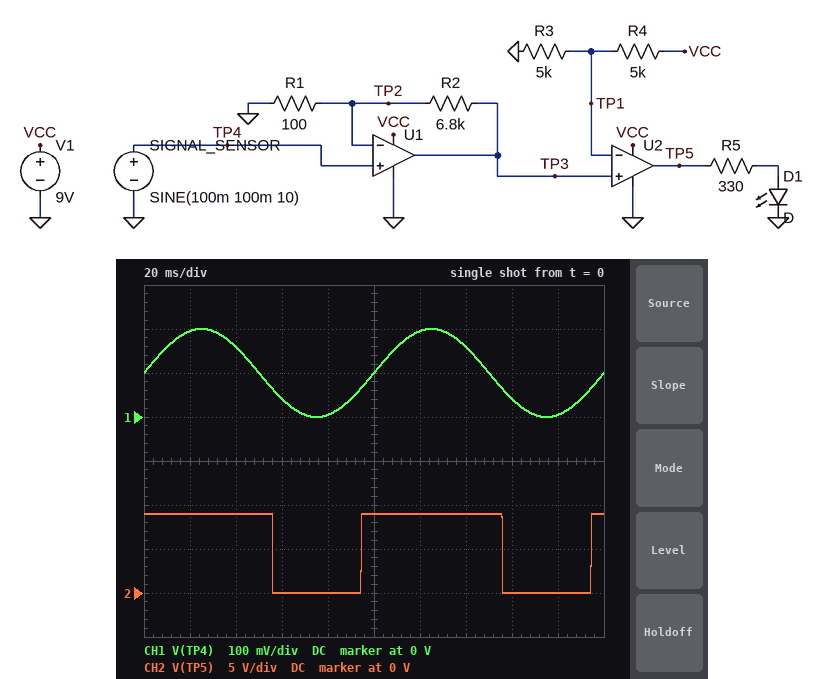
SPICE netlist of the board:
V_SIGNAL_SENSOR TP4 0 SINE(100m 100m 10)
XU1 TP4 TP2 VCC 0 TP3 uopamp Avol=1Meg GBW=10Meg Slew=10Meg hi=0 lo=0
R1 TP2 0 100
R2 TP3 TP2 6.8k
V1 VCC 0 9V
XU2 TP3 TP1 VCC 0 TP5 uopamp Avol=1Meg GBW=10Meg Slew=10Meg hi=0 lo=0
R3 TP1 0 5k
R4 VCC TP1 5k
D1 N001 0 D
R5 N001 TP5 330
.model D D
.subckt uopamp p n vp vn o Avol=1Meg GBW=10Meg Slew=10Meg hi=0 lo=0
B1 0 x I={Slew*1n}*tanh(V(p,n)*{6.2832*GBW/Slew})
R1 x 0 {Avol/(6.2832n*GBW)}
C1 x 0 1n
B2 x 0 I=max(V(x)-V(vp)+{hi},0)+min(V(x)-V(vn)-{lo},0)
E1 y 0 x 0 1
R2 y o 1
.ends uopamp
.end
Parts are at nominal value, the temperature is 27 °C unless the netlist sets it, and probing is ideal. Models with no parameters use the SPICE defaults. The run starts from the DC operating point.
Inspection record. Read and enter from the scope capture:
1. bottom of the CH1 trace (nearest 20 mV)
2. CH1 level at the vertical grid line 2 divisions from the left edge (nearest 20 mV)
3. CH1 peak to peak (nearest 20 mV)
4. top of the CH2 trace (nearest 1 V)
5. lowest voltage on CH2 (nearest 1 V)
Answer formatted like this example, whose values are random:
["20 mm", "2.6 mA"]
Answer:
["0 V", "160 mV", "200 mV", "9 V", "0 V"]
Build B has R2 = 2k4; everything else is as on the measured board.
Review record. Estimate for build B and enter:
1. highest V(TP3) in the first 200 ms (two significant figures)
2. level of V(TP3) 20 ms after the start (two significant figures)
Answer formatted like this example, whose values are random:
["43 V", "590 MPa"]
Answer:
["5.0 V", "4.9 V"]
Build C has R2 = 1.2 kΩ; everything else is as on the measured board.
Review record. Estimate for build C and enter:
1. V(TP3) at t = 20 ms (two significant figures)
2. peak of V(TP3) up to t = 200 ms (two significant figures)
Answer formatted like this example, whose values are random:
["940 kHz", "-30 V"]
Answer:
["2.5 V", "2.6 V"]
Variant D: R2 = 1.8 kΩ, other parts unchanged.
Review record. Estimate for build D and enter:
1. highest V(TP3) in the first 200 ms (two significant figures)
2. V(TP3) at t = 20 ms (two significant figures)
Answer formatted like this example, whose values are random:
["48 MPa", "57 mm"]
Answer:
["3.8 V", "3.7 V"]
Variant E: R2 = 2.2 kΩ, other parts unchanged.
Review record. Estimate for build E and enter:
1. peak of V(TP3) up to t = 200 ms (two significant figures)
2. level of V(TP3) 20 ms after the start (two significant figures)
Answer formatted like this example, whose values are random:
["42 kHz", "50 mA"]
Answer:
["4.6 V", "4.5 V"]
